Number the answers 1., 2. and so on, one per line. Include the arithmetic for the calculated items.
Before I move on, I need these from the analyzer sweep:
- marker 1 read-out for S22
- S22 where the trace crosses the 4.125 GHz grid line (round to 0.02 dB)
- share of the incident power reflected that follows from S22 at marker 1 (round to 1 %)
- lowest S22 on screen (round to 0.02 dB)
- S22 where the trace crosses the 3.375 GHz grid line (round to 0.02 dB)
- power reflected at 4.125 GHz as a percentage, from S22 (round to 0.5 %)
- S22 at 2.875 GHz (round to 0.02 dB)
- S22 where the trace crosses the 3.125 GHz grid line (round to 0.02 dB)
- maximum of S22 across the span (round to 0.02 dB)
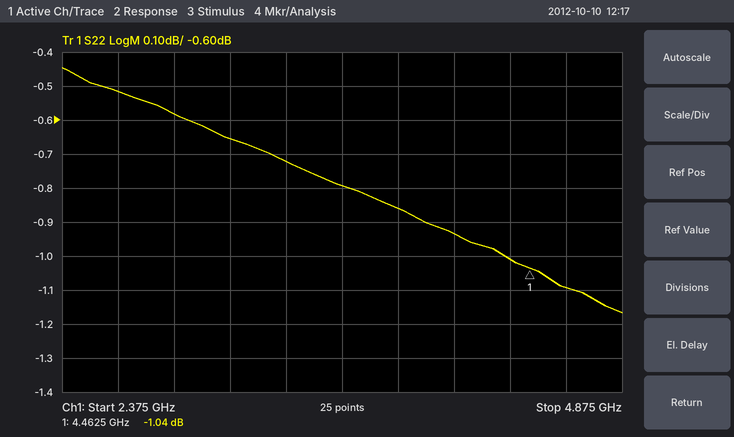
1. -1.04 dB
2. -0.94 dB
3. 10^(-1.04/10) ≈ 79 %
4. -1.16 dB
5. -0.72 dB
6. 10^(-0.94/10) ≈ 80.5 %
7. -0.58 dB
8. -0.66 dB
9. -0.44 dB
